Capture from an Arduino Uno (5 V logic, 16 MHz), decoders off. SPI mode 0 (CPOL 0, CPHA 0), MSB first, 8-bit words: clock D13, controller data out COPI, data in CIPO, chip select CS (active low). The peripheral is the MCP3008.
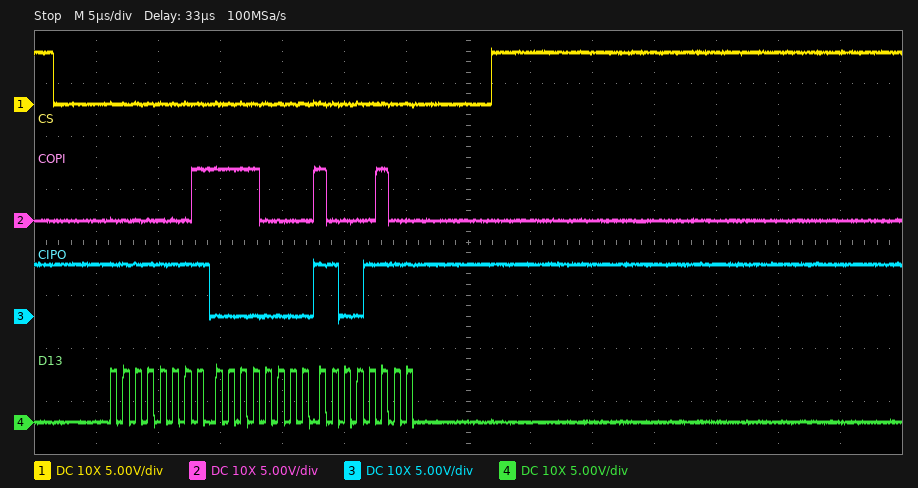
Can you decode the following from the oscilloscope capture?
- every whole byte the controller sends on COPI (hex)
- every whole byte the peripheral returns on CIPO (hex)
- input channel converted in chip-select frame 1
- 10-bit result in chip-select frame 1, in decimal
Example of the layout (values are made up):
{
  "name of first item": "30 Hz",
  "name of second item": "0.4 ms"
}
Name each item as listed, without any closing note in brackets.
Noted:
{
  "every whole byte the controller sends on COPI": "01 F0 84",
  "every whole byte the peripheral returns on CIPO": "FF 00 CF",
  "input channel converted in chip-select frame 1": "7",
  "10-bit result in chip-select frame 1, in decimal": "207"
}
